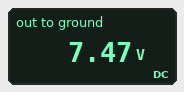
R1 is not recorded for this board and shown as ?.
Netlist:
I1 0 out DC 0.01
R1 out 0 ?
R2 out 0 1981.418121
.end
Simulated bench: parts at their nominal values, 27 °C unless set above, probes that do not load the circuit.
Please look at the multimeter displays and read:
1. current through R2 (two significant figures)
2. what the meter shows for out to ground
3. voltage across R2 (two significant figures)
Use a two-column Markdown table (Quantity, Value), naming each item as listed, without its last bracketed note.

| Quantity | Value |
|---|---|
| current through R2 | 3.8 mA |
| what the meter shows for out to ground | 7.47 V |
| voltage across R2 | 7.5 V |
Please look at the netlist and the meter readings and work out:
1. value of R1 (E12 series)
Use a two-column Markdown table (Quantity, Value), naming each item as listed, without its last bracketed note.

| Quantity | Value |
|---|---|
| value of R1 | 1.2 kΩ |
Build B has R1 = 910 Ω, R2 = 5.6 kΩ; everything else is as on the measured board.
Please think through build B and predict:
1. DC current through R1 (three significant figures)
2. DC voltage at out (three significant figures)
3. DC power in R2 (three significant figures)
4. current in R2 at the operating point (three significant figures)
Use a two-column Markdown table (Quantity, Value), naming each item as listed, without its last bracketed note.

| Quantity | Value |
|---|---|
| DC current through R1 | 8.60 mA |
| DC voltage at out | 7.83 V |
| DC power in R2 | 10.9 mW |
| current in R2 at the operating point | 1.40 mA |
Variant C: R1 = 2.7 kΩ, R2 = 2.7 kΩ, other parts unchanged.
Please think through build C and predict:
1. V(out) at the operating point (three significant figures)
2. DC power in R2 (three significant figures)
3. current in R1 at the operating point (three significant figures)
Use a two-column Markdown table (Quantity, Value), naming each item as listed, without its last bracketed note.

| Quantity | Value |
|---|---|
| V(out) at the operating point | 13.5 V |
| DC power in R2 | 67.5 mW |
| current in R1 at the operating point | 5.00 mA |
